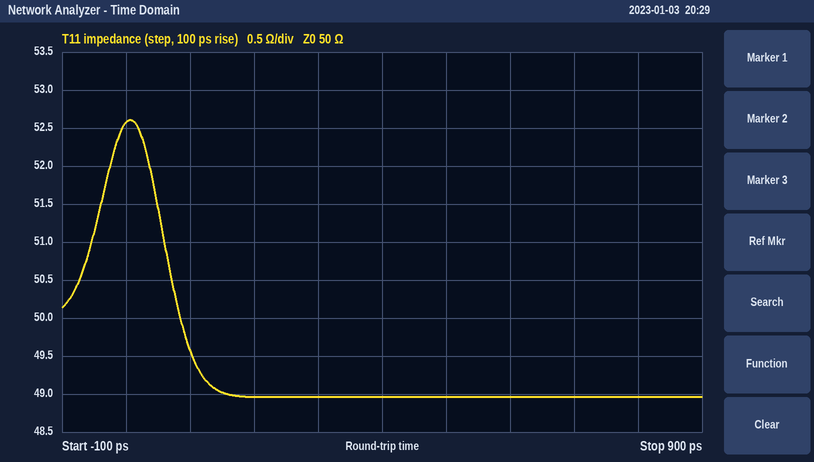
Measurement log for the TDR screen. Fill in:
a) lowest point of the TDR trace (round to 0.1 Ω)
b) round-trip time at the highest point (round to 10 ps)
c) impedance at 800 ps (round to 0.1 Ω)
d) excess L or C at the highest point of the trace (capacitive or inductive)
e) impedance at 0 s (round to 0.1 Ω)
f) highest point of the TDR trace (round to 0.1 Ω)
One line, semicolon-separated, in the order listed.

49.0 Ω; 10 ps; 49.0 Ω; inductive; 52.6 Ω; 52.6 Ω
